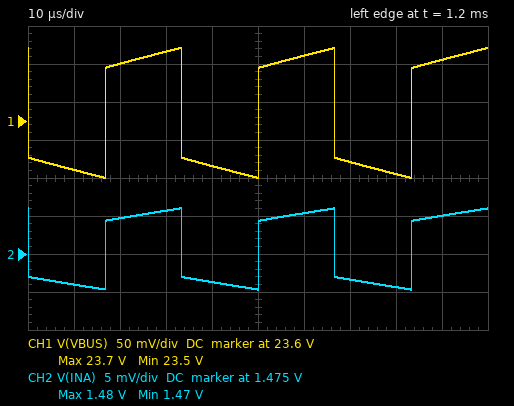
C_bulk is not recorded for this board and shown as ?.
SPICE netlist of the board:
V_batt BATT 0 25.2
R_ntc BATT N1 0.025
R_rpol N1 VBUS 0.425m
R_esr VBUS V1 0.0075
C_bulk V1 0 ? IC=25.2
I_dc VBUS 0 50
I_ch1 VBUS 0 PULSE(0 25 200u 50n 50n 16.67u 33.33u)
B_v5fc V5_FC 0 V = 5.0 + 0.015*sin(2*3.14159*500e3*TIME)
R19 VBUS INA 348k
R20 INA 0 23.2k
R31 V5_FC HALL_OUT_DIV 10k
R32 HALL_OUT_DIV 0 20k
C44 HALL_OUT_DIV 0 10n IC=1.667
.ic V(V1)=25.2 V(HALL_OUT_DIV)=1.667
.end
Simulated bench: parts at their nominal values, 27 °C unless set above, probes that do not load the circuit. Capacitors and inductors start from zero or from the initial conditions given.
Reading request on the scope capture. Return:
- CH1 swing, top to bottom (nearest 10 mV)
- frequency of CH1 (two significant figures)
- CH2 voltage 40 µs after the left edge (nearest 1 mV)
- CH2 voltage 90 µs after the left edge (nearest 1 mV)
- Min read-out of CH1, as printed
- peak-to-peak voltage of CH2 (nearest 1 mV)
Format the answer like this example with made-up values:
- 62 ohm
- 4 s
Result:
- 170 mV
- 30 kHz
- 1.471 V
- 1.480 V
- 23.5 V
- 11 mV
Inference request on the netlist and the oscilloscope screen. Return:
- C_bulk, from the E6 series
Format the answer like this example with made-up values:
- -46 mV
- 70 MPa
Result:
- 4.7 mF
